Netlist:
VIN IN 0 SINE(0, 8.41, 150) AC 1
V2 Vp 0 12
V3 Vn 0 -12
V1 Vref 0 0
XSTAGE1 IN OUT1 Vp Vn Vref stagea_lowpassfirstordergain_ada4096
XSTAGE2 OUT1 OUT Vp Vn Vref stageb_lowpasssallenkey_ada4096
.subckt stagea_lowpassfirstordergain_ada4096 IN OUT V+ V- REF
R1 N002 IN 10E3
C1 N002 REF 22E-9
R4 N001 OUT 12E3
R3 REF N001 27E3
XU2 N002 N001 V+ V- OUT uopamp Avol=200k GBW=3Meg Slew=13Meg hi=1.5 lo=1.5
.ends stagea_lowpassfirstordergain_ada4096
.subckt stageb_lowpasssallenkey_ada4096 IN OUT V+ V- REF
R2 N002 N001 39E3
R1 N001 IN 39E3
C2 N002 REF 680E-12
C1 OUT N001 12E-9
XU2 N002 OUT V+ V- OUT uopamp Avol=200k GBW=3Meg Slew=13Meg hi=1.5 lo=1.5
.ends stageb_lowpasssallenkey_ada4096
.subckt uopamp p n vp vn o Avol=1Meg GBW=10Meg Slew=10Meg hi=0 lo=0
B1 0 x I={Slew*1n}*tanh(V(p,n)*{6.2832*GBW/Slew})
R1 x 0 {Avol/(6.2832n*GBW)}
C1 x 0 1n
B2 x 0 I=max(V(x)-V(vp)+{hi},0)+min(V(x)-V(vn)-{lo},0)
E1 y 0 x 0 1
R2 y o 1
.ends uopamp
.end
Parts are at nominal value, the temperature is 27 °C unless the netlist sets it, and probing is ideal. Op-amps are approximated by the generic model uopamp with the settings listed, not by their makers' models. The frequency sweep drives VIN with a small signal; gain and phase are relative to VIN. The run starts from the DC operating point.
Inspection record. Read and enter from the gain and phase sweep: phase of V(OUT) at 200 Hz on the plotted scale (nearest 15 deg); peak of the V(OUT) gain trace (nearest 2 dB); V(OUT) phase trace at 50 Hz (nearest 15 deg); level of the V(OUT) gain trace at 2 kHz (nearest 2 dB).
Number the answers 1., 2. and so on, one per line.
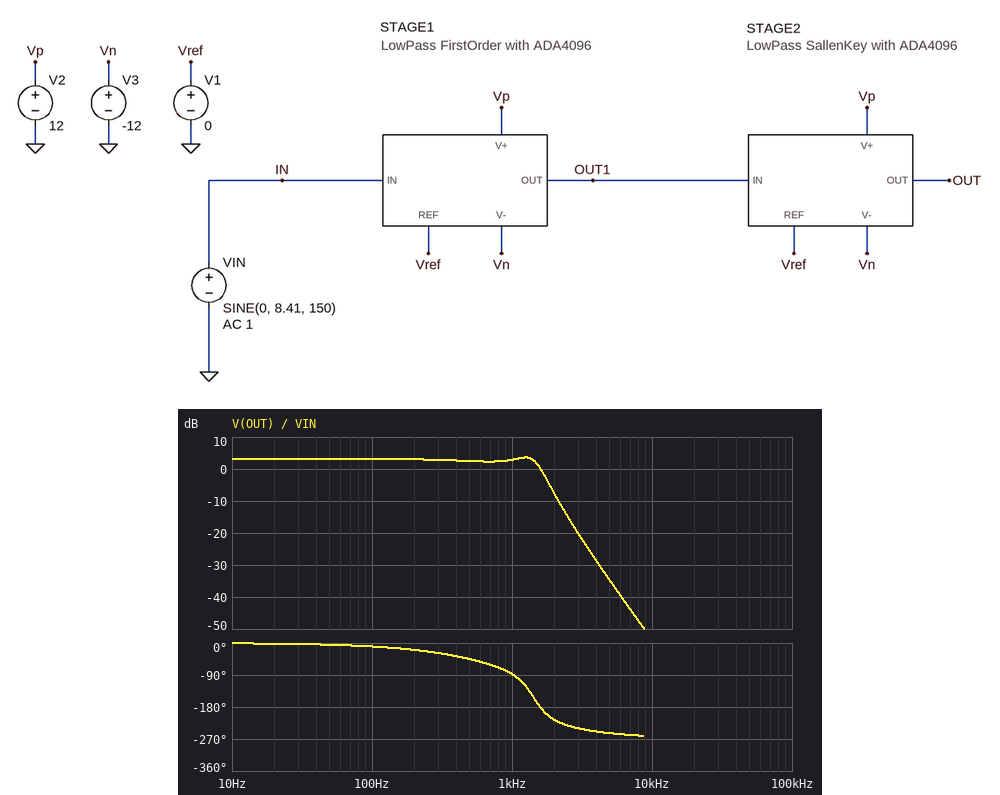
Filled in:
1. -15 deg
2. 4 dB
3. 0 deg
4. -8 dB
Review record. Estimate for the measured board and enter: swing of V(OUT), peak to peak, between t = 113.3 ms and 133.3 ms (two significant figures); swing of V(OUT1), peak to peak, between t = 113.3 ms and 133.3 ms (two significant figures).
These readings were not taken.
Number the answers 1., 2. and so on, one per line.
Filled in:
1. 21 V
2. 21 V
